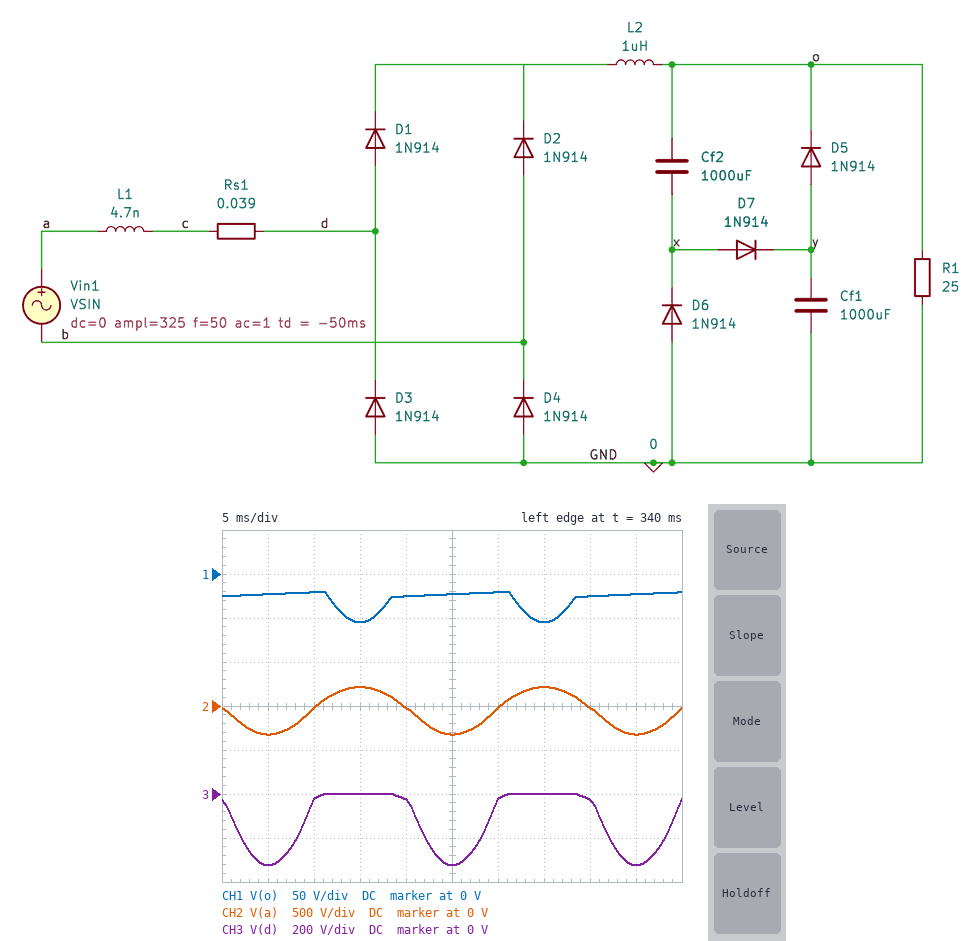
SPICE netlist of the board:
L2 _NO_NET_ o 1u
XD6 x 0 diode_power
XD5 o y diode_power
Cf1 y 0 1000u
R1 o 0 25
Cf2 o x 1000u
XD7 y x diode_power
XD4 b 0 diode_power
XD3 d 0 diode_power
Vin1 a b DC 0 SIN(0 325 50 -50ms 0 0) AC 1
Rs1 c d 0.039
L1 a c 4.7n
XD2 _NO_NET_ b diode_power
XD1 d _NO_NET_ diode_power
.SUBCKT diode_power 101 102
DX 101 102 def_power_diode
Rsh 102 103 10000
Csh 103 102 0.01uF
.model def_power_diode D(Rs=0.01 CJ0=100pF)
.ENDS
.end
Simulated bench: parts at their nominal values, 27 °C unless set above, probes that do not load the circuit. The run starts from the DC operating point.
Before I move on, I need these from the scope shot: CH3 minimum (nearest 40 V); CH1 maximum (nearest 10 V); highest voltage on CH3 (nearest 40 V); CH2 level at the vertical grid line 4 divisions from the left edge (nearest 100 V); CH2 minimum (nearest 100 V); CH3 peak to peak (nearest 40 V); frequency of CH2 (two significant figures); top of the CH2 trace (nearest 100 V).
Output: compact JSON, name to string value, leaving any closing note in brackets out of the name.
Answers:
{"CH3 minimum": "-320 V", "CH1 maximum": "-20 V", "highest voltage on CH3": "0 V", "CH2 level at the vertical grid line 4 divisions from the left edge": "0 V", "CH2 minimum": "-300 V", "CH3 peak to peak": "320 V", "frequency of CH2": "50 Hz", "top of the CH2 trace": "200 V"}
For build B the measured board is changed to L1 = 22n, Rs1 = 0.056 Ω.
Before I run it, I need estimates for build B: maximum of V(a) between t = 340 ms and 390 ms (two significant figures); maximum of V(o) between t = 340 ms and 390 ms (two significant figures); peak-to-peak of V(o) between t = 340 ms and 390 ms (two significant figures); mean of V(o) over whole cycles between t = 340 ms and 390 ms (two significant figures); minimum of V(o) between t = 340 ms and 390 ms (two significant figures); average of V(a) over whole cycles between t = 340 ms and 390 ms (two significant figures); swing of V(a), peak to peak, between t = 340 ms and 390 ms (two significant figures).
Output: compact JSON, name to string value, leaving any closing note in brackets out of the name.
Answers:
{"maximum of V(a) between t = 340 ms and 390 ms": "240 V", "maximum of V(o) between t = 340 ms and 390 ms": "-16 V", "peak-to-peak of V(o) between t = 340 ms and 390 ms": "27 V", "mean of V(o) over whole cycles between t = 340 ms and 390 ms": "-24 V", "minimum of V(o) between t = 340 ms and 390 ms": "-43 V", "average of V(a) over whole cycles between t = 340 ms and 390 ms": "-31 V", "swing of V(a), peak to peak, between t = 340 ms and 390 ms": "560 V"}
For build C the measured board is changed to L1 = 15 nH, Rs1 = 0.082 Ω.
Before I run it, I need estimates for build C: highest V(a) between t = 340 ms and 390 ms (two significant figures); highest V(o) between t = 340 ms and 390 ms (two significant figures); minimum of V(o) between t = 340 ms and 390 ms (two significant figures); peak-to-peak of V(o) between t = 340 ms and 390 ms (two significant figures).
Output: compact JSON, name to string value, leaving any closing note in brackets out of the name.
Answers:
{"highest V(a) between t = 340 ms and 390 ms": "260 V", "highest V(o) between t = 340 ms and 390 ms": "-11 V", "minimum of V(o) between t = 340 ms and 390 ms": "-32 V", "peak-to-peak of V(o) between t = 340 ms and 390 ms": "20 V"}
